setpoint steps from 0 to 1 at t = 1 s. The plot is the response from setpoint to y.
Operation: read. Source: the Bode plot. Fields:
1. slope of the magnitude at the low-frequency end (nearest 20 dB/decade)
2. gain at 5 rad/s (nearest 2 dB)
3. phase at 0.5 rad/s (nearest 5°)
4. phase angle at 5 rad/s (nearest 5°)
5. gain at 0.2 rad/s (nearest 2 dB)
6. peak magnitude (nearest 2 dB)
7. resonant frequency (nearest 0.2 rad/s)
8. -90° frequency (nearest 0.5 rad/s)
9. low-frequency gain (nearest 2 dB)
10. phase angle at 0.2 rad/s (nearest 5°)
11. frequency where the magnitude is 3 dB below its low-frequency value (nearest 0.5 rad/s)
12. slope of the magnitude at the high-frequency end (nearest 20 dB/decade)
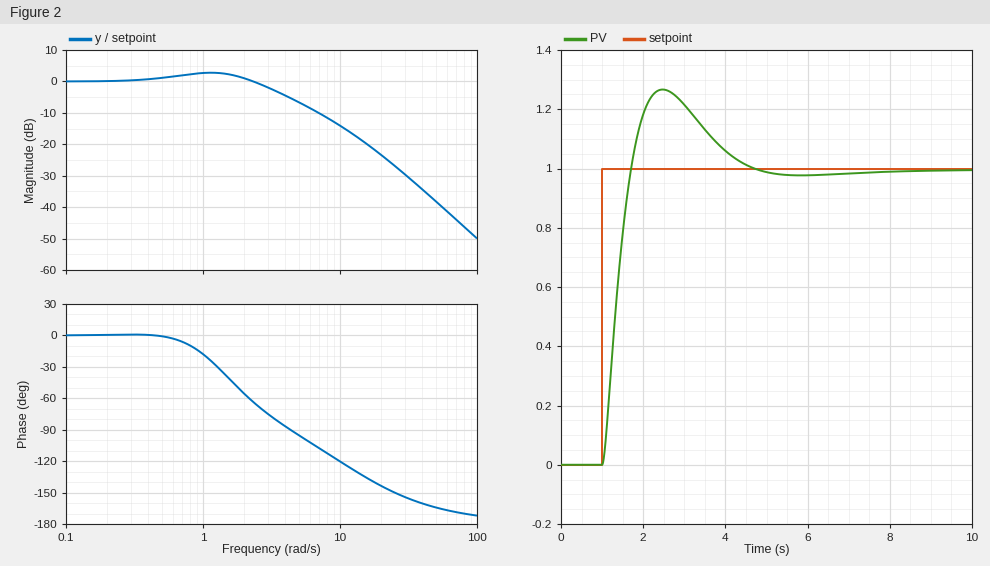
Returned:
0 dB/decade
-6 dB
0°
-95°
0 dB
2 dB
1.2 rad/s
4.5 rad/s
0 dB
0°
3.5 rad/s
-40 dB/decade
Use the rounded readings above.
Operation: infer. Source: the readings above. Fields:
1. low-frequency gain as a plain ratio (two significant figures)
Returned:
1.0
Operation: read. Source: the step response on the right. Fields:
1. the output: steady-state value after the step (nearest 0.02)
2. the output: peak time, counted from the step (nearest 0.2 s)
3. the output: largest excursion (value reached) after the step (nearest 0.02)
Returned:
1.00
1.4 s
1.26
